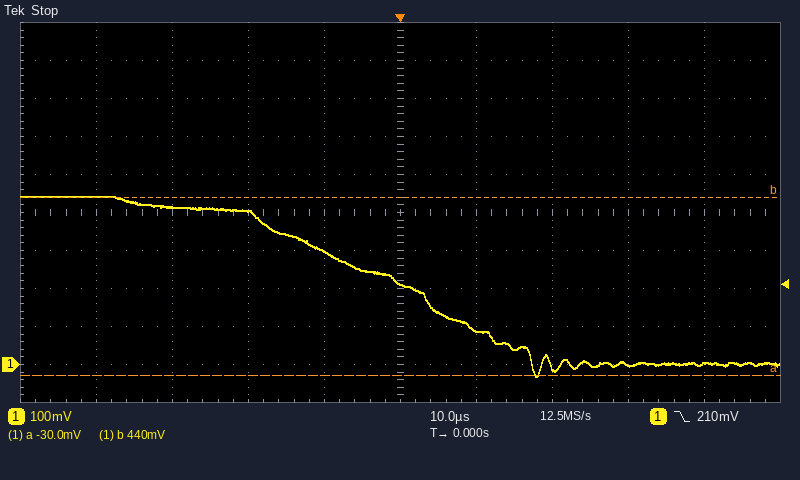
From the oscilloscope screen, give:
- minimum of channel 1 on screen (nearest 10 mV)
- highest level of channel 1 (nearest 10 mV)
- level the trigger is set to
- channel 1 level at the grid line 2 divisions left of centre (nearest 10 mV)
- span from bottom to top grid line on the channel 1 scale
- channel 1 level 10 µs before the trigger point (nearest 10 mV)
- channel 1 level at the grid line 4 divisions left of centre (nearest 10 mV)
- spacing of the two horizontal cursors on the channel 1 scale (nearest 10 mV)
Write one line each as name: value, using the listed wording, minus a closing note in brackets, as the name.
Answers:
minimum of channel 1 on screen: -30 mV
highest level of channel 1: 440 mV
level the trigger is set to: 210 mV
channel 1 level at the grid line 2 divisions left of centre: 400 mV
span from bottom to top grid line on the channel 1 scale: 1 V
channel 1 level 10 µs before the trigger point: 300 mV
channel 1 level at the grid line 4 divisions left of centre: 440 mV
spacing of the two horizontal cursors on the channel 1 scale: 470 mV
